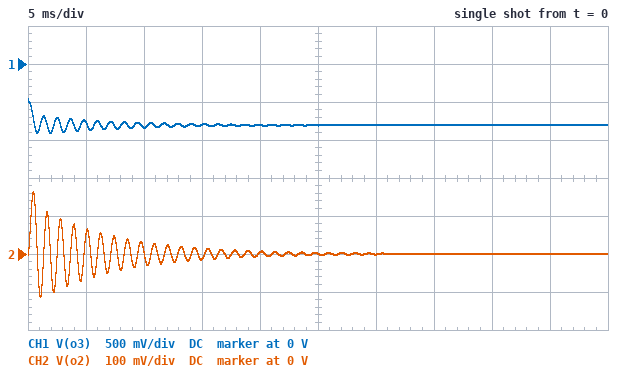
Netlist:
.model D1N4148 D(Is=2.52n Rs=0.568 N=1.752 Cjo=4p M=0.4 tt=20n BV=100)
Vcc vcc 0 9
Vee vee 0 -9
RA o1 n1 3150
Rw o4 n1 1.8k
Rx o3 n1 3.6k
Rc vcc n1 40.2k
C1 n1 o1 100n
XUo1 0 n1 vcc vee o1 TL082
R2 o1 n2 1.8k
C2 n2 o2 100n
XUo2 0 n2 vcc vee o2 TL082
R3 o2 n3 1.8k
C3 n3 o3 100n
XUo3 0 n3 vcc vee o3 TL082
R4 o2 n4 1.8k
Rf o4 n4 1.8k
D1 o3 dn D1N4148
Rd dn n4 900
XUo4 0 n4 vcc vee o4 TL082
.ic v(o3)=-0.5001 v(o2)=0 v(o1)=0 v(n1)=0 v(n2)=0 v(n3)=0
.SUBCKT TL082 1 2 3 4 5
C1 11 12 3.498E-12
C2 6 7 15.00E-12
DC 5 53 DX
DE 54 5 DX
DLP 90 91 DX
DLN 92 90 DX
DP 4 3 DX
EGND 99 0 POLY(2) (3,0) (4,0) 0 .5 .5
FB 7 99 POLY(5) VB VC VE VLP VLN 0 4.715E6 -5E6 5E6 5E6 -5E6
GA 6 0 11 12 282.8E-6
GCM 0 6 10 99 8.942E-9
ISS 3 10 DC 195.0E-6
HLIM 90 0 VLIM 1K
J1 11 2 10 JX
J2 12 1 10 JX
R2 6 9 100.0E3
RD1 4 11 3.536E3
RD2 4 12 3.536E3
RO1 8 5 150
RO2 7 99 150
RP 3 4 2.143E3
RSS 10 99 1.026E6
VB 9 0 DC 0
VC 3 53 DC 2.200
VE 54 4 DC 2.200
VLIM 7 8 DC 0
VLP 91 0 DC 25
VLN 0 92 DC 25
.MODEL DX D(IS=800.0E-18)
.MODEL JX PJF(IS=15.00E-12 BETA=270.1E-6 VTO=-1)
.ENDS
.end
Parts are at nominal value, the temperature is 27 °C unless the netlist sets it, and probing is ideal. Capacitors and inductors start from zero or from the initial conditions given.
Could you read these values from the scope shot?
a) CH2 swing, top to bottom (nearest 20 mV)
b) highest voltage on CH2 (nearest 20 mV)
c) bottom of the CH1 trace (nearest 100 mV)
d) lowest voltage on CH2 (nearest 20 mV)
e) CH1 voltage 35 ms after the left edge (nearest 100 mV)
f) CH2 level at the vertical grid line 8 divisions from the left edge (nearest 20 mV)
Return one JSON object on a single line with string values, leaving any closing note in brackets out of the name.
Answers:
{"CH2 swing, top to bottom": "280 mV", "highest voltage on CH2": "160 mV", "bottom of the CH1 trace": "-900 mV", "lowest voltage on CH2": "-120 mV", "CH1 voltage 35 ms after the left edge": "-800 mV", "CH2 level at the vertical grid line 8 divisions from the left edge": "0 V"}
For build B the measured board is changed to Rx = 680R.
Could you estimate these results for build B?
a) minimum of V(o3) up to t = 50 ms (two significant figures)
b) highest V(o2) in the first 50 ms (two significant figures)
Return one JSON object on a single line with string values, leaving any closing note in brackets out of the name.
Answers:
{"minimum of V(o3) up to t = 50 ms": "-7.5 V", "highest V(o2) in the first 50 ms": "7.5 V"}
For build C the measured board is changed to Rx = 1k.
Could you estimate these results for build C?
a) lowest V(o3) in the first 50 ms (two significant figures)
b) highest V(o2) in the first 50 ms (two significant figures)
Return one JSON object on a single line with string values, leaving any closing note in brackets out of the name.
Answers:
{"lowest V(o3) in the first 50 ms": "-7.5 V", "highest V(o2) in the first 50 ms": "7.5 V"}
